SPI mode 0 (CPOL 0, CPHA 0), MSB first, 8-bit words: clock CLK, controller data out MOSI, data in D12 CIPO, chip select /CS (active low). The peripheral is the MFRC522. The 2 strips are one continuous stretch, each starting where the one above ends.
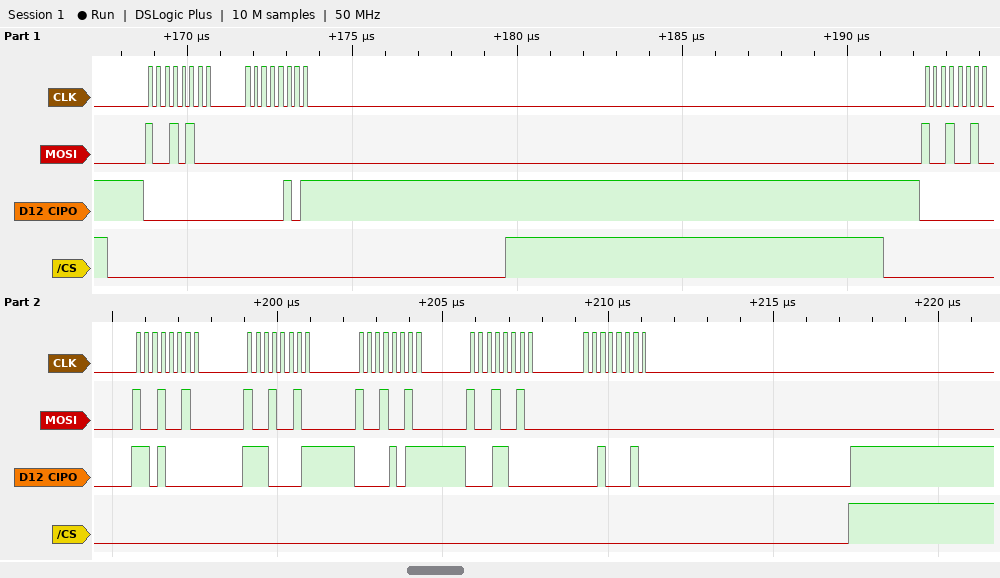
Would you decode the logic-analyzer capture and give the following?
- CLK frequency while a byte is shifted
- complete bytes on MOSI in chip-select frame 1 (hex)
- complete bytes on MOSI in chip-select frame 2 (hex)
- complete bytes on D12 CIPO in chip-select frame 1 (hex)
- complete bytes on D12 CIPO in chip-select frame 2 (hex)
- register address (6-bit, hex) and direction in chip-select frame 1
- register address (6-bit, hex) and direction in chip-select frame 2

4 MHz
94 00
92 92 92 92 92 00
00 05
00 D0 E1 0B 18 22
0x0A read
0x09 read
